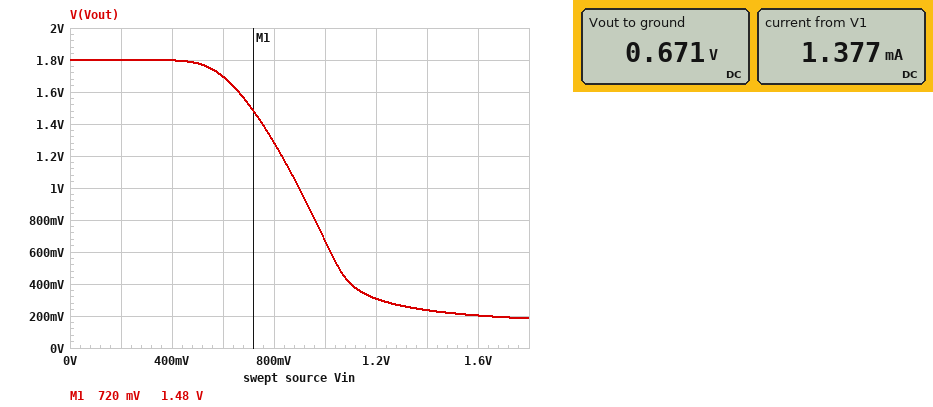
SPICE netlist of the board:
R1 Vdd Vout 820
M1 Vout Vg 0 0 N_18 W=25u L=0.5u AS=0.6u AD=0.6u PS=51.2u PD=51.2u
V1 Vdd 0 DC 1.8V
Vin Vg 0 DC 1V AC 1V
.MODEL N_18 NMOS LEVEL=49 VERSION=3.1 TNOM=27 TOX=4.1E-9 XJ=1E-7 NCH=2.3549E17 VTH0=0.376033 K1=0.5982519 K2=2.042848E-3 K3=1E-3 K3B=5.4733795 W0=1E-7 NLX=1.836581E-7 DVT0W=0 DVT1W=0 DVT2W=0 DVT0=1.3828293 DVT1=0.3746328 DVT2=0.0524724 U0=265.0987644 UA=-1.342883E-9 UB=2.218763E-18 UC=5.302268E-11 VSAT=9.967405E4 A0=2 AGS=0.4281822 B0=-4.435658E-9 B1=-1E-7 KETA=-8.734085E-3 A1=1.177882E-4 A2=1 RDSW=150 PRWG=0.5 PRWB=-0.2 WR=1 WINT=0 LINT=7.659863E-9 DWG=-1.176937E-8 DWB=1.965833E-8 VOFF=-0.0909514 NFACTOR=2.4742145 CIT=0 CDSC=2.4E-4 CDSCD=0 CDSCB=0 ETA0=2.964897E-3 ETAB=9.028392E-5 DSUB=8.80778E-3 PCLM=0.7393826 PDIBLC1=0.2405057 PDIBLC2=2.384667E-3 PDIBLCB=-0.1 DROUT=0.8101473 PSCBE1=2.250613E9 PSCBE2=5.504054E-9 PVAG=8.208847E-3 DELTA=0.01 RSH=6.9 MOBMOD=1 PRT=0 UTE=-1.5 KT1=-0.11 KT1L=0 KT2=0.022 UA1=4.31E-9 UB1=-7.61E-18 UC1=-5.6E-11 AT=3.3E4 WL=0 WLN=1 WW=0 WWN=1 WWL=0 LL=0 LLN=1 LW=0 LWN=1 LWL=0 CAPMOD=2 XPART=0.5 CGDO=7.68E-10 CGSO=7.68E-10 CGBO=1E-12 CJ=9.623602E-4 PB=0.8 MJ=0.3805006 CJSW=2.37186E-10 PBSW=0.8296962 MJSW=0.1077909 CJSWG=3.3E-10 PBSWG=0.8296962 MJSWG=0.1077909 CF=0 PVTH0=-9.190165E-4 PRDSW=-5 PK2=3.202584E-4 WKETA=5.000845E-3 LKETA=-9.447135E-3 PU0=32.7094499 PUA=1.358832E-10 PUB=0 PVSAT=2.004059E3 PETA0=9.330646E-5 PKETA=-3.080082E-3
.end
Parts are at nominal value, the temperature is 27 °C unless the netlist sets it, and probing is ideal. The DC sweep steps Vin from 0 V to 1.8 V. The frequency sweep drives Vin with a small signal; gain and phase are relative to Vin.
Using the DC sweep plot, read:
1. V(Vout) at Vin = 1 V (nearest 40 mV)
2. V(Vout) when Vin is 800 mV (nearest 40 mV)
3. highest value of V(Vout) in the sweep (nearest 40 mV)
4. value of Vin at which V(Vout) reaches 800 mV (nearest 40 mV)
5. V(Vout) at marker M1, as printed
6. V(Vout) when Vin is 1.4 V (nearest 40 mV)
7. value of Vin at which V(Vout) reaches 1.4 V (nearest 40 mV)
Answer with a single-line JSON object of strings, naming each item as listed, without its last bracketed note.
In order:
{"V(Vout) at Vin = 1 V": "680 mV", "V(Vout) when Vin is 800 mV": "1.28 V", "highest value of V(Vout) in the sweep": "1.80 V", "value of Vin at which V(Vout) reaches 800 mV": "960 mV", "V(Vout) at marker M1, as printed": "1.48 V", "V(Vout) when Vin is 1.4 V": "240 mV", "value of Vin at which V(Vout) reaches 1.4 V": "760 mV"}
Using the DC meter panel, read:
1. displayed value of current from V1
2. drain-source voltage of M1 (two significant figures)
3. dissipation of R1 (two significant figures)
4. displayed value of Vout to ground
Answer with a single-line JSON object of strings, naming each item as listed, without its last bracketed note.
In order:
{"displayed value of current from V1": "1.377 mA", "drain-source voltage of M1": "670 mV", "dissipation of R1": "1.6 mW", "displayed value of Vout to ground": "0.671 V"}
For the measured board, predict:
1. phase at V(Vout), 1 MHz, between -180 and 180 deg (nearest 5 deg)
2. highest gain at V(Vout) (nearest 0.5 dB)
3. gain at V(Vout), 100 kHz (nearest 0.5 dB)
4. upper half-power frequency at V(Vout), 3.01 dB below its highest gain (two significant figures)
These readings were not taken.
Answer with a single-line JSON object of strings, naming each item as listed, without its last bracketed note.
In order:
{"phase at V(Vout), 1 MHz, between -180 and 180 deg": "115 deg", "highest gain at V(Vout)": "10.5 dB", "gain at V(Vout), 100 kHz": "10.0 dB", "upper half-power frequency at V(Vout), 3.01 dB below its highest gain": "460 kHz"}
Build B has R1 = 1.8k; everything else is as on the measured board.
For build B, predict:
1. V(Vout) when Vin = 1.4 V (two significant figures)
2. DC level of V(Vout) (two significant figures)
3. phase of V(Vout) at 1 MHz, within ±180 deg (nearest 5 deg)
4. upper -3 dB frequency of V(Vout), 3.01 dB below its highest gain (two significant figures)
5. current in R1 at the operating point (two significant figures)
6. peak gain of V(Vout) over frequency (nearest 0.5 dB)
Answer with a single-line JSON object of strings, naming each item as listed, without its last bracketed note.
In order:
{"V(Vout) when Vin = 1.4 V": "100 mV", "DC level of V(Vout)": "180 mV", "phase of V(Vout) at 1 MHz, within ±180 deg": "140 deg", "upper -3 dB frequency of V(Vout), 3.01 dB below its highest gain": "1.2 MHz", "current in R1 at the operating point": "900 µA", "peak gain of V(Vout) over frequency": "-6.5 dB"}
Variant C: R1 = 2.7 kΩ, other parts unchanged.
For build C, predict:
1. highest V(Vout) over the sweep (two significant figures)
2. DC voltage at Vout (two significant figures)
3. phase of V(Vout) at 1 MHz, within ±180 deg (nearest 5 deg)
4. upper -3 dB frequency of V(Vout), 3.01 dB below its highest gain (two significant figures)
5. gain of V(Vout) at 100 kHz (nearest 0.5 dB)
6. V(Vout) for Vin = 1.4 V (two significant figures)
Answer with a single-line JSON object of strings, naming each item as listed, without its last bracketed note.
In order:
{"highest V(Vout) over the sweep": "1.8 V", "DC voltage at Vout": "110 mV", "phase of V(Vout) at 1 MHz, within ±180 deg": "145 deg", "upper -3 dB frequency of V(Vout), 3.01 dB below its highest gain": "1.5 MHz", "gain of V(Vout) at 100 kHz": "-12.5 dB", "V(Vout) for Vin = 1.4 V": "69 mV"}
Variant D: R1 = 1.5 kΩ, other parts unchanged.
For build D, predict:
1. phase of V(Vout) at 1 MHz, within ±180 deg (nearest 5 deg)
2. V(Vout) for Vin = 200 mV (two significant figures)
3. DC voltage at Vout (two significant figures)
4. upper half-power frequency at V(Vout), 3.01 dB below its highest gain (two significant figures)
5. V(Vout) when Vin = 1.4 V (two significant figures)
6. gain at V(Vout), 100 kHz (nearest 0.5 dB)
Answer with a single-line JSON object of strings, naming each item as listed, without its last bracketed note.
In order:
{"phase of V(Vout) at 1 MHz, within ±180 deg": "135 deg", "V(Vout) for Vin = 200 mV": "1.8 V", "DC voltage at Vout": "230 mV", "upper half-power frequency at V(Vout), 3.01 dB below its highest gain": "1.0 MHz", "V(Vout) when Vin = 1.4 V": "130 mV", "gain at V(Vout), 100 kHz": "-3.0 dB"}
